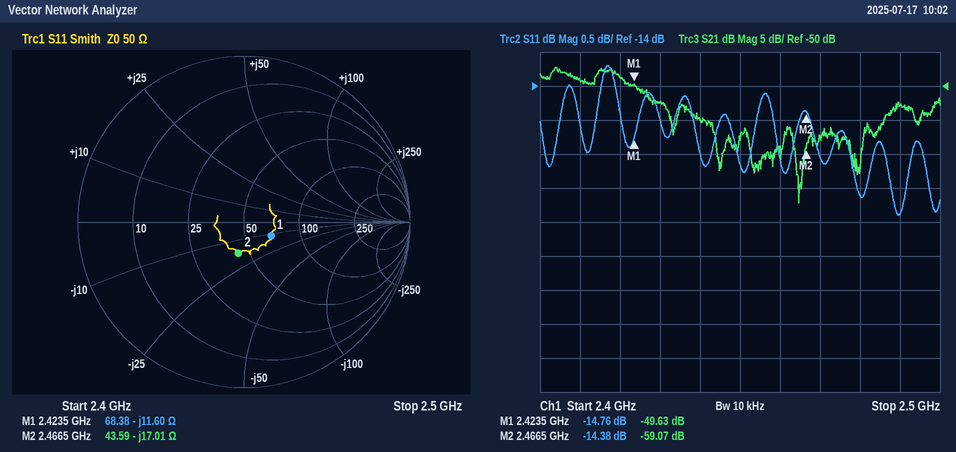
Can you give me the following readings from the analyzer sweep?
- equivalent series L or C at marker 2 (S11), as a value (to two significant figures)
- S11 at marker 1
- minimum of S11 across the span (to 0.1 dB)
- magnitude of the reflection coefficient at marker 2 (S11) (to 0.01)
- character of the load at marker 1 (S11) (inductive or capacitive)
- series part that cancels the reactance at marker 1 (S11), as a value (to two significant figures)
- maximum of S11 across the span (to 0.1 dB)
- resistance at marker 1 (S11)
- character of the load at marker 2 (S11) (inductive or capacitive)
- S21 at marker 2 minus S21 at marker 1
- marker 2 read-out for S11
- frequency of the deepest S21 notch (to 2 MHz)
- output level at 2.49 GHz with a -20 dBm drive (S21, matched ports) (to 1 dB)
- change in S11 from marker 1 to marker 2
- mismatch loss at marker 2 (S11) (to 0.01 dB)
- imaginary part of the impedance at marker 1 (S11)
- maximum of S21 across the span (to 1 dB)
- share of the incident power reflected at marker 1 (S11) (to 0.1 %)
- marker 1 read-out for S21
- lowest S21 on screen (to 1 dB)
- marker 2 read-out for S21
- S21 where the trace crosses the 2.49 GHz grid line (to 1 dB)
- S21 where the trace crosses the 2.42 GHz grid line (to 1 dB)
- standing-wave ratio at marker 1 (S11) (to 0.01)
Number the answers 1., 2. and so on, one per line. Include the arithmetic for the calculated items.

1. C = 1/(2π × 2.4665 GHz × 17.01 Ω) ≈ 3.8 pF
2. -14.76 dB
3. -15.9 dB
4. 0.19
5. capacitive
6. L = 11.6 Ω/(2π × 2.4235 GHz) ≈ 762 pH, so 760 pH to two significant figures
7. -13.7 dB
8. 68.38 Ω
9. capacitive
10. -59.07 − (-49.63) = -9.44 dB
11. -14.38 dB
12. 2.464 GHz
13. -20 dBm + (-53 dB) = -73 dBm
14. -14.38 − (-14.76) = 0.38 dB
15. −10 log10(1 − 10^(-14.38/10)) ≈ 0.16 dB
16. -11.60 Ω
17. -47 dB
18. 10^(-14.76/10) ≈ 3.3 %
19. -49.63 dB
20. -67 dB
21. -59.07 dB
22. -53 dB
23. -49 dB
24. 1.45
